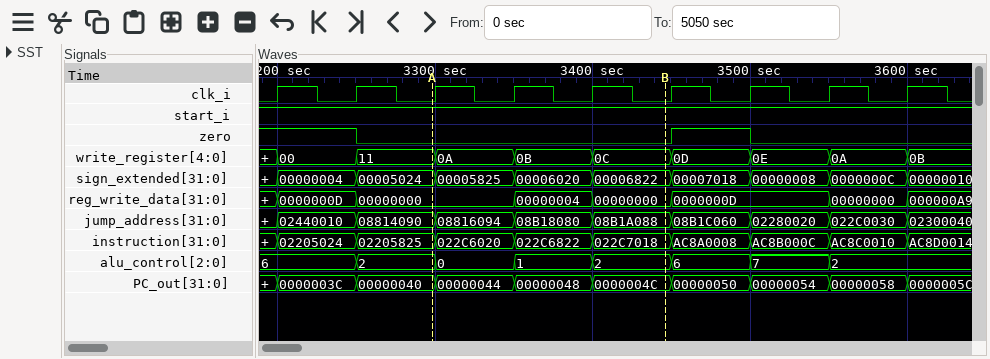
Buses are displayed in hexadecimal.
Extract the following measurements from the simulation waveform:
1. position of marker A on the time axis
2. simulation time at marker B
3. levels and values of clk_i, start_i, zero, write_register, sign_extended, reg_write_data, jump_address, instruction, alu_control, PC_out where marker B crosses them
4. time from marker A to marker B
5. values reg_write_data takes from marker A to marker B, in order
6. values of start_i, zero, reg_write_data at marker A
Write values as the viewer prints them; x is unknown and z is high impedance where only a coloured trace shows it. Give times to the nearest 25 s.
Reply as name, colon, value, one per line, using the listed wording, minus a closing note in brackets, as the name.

position of marker A on the time axis: 3300 s
simulation time at marker B: 3450 s
levels and values of clk_i, start_i, zero, write_register, sign_extended, reg_write_data, jump_address, instruction, alu_control, PC_out where marker B crosses them: clk_i=0, start_i=1, zero=0, write_register=0C, sign_extended=00006822, reg_write_data=00000000, jump_address=08B1A088, instruction=022C7018, alu_control=2, PC_out=0000004C
time from marker A to marker B: 150 s
values reg_write_data takes from marker A to marker B, in order: 00000000, 00000004, 00000000
values of start_i, zero, reg_write_data at marker A: start_i=1, zero=0, reg_write_data=00000000
